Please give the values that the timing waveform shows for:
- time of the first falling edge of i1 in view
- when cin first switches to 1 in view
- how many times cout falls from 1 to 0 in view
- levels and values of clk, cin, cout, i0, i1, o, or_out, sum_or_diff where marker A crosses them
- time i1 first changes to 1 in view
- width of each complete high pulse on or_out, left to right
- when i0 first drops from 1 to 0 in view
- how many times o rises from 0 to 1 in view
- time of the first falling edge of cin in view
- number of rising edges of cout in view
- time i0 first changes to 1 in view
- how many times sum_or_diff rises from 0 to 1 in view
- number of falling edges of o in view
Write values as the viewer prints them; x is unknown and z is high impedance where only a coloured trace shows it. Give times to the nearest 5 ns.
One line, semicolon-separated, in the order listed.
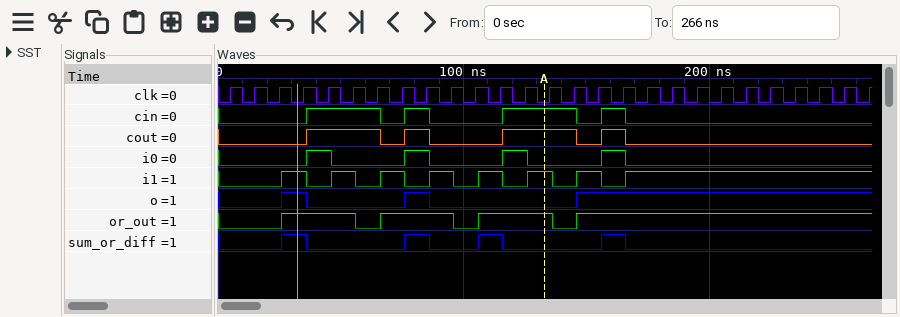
35 ns; 35 ns; 4; clk=0, cin=1, cout=1, i0=0, i1=1, o=0, or_out=1, sum_or_diff=0; 25 ns; 30 ns, 30 ns, 30 ns; 45 ns; 3; 65 ns; 4; 35 ns; 4; 2
